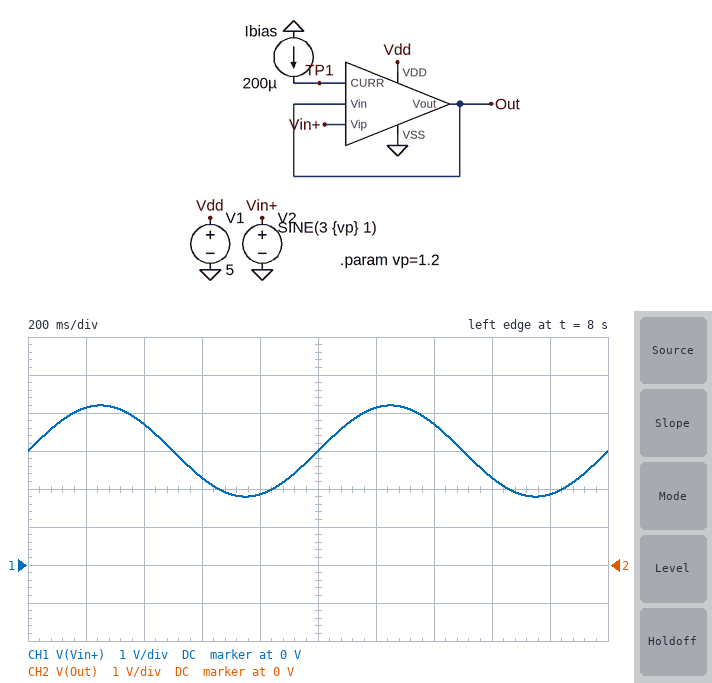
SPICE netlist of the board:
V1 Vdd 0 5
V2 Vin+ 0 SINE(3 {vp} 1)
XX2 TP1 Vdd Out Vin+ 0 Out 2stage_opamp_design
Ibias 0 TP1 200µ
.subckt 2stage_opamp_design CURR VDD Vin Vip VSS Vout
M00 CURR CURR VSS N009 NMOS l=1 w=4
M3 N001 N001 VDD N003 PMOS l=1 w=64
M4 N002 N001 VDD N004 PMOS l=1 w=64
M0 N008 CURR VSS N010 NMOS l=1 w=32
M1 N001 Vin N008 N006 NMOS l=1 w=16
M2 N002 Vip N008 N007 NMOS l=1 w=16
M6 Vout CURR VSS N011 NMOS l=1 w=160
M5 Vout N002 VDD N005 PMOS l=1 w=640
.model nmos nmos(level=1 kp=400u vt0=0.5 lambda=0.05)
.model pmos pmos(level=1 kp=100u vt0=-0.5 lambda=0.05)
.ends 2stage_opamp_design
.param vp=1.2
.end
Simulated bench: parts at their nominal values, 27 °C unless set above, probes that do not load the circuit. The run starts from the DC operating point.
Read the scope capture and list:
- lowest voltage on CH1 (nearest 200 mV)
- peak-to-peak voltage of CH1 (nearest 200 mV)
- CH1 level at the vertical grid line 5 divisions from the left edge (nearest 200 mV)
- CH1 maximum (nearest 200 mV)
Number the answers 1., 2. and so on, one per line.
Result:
1. 1.8 V
2. 2.4 V
3. 3.0 V
4. 4.2 V
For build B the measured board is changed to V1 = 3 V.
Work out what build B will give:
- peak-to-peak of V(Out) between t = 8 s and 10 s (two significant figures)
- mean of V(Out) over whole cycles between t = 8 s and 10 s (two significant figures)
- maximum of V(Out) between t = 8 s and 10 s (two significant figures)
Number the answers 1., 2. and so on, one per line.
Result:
1. 980 mV
2. 2.5 V
3. 2.8 V
